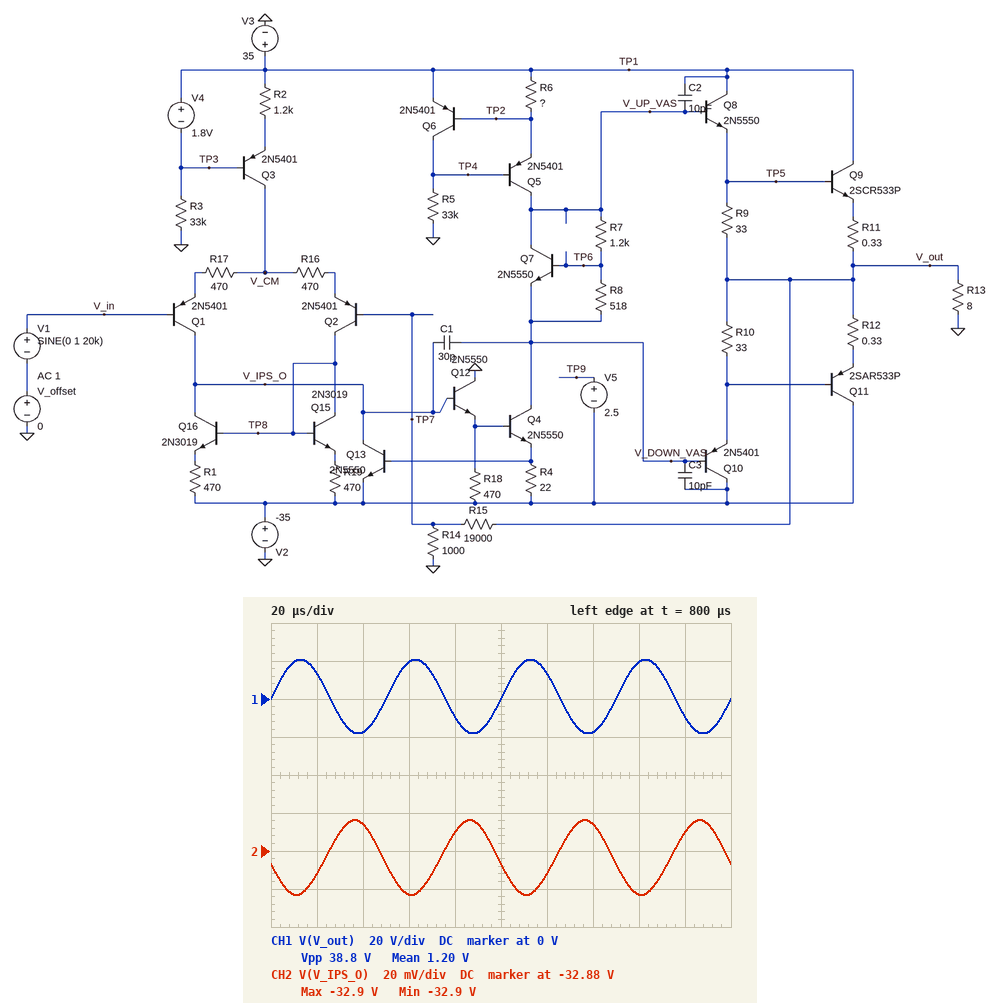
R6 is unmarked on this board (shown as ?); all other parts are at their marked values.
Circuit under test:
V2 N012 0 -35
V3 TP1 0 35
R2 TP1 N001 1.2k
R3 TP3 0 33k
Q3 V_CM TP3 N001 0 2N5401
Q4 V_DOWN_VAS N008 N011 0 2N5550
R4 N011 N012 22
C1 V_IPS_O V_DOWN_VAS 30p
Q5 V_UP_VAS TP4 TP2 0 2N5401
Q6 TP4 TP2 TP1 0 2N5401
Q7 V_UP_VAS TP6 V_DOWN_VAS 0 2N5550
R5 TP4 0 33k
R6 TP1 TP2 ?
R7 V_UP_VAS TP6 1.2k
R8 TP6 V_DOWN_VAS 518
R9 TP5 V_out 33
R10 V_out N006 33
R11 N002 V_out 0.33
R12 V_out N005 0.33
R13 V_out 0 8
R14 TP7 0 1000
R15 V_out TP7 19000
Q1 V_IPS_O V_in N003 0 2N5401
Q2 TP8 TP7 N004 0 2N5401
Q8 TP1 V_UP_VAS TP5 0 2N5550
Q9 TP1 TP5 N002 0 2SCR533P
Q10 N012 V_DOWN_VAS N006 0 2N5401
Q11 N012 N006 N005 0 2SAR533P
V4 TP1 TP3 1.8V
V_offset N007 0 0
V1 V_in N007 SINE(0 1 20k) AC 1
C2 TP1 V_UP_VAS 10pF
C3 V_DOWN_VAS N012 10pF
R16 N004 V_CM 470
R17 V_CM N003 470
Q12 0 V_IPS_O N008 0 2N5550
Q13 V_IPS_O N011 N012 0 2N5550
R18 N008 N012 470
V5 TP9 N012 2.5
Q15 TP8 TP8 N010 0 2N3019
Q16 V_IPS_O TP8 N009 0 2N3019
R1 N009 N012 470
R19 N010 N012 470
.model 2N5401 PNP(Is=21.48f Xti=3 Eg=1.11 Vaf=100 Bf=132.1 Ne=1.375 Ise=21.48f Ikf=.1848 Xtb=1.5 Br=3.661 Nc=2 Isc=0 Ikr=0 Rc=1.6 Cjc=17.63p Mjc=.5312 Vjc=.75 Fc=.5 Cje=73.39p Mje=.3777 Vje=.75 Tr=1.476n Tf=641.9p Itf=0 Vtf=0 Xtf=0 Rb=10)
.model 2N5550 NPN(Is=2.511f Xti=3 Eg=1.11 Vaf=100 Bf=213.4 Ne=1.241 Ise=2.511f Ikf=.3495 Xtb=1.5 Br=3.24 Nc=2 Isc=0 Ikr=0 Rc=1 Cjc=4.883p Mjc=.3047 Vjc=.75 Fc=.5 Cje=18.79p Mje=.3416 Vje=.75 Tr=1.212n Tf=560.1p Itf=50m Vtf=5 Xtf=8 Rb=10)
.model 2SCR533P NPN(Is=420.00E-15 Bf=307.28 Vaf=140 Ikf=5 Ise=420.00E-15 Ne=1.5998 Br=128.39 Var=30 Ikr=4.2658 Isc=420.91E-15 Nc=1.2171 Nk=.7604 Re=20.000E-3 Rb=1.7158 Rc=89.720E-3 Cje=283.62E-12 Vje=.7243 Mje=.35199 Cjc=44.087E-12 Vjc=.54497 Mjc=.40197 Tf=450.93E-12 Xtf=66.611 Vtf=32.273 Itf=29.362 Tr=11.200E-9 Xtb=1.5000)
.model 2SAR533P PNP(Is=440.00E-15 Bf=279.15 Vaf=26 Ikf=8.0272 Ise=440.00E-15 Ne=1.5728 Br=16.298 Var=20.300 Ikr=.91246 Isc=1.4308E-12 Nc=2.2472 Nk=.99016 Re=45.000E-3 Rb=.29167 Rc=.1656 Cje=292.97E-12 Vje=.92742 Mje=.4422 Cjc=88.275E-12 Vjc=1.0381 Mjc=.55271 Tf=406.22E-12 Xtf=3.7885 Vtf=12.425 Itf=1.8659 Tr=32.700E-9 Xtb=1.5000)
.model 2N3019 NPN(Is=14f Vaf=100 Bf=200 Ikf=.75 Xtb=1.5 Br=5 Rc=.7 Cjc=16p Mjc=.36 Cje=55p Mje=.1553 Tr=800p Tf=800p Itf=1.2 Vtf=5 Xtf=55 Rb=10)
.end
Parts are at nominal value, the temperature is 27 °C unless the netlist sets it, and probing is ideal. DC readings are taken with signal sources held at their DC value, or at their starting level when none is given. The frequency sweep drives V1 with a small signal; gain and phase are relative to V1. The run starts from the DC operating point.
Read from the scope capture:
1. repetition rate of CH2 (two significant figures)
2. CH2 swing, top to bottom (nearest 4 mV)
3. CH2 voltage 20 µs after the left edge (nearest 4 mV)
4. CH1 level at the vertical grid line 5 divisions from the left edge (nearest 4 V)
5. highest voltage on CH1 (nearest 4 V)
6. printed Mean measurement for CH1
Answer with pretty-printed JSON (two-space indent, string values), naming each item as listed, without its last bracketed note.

{
  "repetition rate of CH2": "20 kHz",
  "CH2 swing, top to bottom": "40 mV",
  "CH2 voltage 20 µs after the left edge": "-32.892 V",
  "CH1 level at the vertical grid line 5 divisions from the left edge": "0 V",
  "highest voltage on CH1": "20 V",
  "printed Mean measurement for CH1": "1.20 V"
}
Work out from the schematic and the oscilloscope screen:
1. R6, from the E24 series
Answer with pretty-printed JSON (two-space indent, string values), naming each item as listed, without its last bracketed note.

{
  "R6, from the E24 series": "22 Ω"
}
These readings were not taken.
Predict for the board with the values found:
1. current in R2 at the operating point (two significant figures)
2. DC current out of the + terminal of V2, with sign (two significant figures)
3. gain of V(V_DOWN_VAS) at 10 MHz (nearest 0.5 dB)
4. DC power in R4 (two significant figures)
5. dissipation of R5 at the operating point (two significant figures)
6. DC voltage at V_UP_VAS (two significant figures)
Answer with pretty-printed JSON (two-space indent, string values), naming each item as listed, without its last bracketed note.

{
  "current in R2 at the operating point": "980 µA",
  "DC current out of the + terminal of V2, with sign": "-73 mA",
  "gain of V(V_DOWN_VAS) at 10 MHz": "-6.5 dB",
  "DC power in R4": "18 mW",
  "dissipation of R5 at the operating point": "34 mW",
  "DC voltage at V_UP_VAS": "2.7 V"
}
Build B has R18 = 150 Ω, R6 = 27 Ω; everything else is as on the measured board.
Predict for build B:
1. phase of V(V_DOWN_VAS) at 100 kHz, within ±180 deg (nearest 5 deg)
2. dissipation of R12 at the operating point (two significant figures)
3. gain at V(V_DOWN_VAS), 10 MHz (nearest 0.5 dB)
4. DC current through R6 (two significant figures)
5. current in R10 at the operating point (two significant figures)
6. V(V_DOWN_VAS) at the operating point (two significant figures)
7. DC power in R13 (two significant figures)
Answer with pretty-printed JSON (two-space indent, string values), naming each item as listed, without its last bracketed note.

{
  "phase of V(V_DOWN_VAS) at 100 kHz, within ±180 deg": "-10 deg",
  "dissipation of R12 at the operating point": "60 µW",
  "gain at V(V_DOWN_VAS), 10 MHz": "-5.0 dB",
  "DC current through R6": "23 mA",
  "current in R10 at the operating point": "18 mA",
  "V(V_DOWN_VAS) at the operating point": "-800 mV",
  "DC power in R13": "33 mW"
}
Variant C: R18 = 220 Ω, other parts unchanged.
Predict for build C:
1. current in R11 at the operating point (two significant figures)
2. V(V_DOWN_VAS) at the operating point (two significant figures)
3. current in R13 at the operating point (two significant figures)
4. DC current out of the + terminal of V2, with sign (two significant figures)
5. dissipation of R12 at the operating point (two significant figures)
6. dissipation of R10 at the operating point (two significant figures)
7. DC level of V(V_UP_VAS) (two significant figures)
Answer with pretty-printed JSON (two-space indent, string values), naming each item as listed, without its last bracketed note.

{
  "current in R11 at the operating point": "180 mA",
  "V(V_DOWN_VAS) at the operating point": "50 mV",
  "current in R13 at the operating point": "170 mA",
  "DC current out of the + terminal of V2, with sign": "-70 mA",
  "dissipation of R12 at the operating point": "81 µW",
  "dissipation of R10 at the operating point": "11 mW",
  "DC level of V(V_UP_VAS)": "2.9 V"
}
